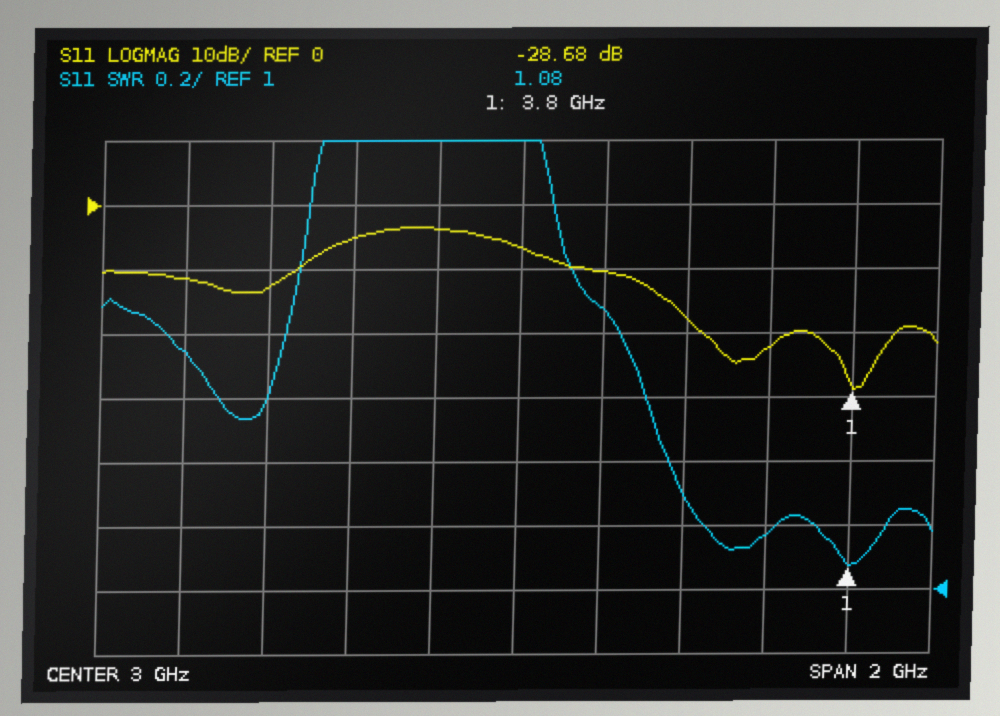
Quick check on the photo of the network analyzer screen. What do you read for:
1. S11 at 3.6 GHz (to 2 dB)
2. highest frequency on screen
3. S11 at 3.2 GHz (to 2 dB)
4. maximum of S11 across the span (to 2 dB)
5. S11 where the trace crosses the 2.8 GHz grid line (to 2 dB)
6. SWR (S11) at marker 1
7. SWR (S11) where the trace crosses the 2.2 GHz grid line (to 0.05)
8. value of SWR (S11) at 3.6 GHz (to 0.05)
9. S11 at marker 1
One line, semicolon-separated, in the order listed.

-22 dB; 4 GHz; -10 dB; -4 dB; -4 dB; 1.08; 1.75; 1.15; -28.68 dB
